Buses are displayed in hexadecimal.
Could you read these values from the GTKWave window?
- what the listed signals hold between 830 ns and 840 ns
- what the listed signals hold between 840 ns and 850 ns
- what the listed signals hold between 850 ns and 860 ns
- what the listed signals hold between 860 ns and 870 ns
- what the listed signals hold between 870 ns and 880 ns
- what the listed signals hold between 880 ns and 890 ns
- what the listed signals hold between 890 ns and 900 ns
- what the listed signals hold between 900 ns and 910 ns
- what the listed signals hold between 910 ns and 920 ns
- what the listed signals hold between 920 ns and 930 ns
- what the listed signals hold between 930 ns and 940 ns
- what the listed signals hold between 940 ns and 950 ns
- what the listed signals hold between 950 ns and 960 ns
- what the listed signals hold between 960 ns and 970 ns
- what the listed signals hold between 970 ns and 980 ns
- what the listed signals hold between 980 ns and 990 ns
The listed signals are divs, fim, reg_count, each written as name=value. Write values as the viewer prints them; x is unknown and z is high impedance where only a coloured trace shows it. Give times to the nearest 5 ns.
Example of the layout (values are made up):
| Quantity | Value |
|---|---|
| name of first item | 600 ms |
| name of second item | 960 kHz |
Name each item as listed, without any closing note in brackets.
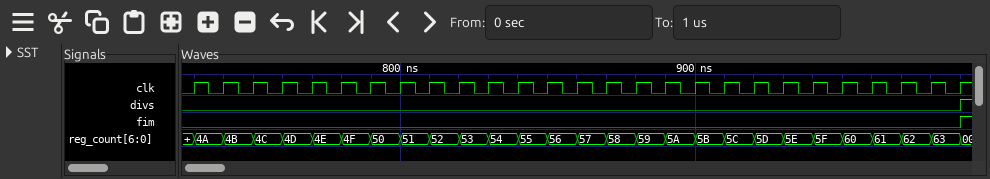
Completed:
| Quantity | Value |
|---|---|
| what the listed signals hold between 830 ns and 840 ns | divs=0, fim=0, reg_count=54 |
| what the listed signals hold between 840 ns and 850 ns | divs=0, fim=0, reg_count=55 |
| what the listed signals hold between 850 ns and 860 ns | divs=0, fim=0, reg_count=56 |
| what the listed signals hold between 860 ns and 870 ns | divs=0, fim=0, reg_count=57 |
| what the listed signals hold between 870 ns and 880 ns | divs=0, fim=0, reg_count=58 |
| what the listed signals hold between 880 ns and 890 ns | divs=0, fim=0, reg_count=59 |
| what the listed signals hold between 890 ns and 900 ns | divs=0, fim=0, reg_count=5A |
| what the listed signals hold between 900 ns and 910 ns | divs=0, fim=0, reg_count=5B |
| what the listed signals hold between 910 ns and 920 ns | divs=0, fim=0, reg_count=5C |
| what the listed signals hold between 920 ns and 930 ns | divs=0, fim=0, reg_count=5D |
| what the listed signals hold between 930 ns and 940 ns | divs=0, fim=0, reg_count=5E |
| what the listed signals hold between 940 ns and 950 ns | divs=0, fim=0, reg_count=5F |
| what the listed signals hold between 950 ns and 960 ns | divs=0, fim=0, reg_count=60 |
| what the listed signals hold between 960 ns and 970 ns | divs=0, fim=0, reg_count=61 |
| what the listed signals hold between 970 ns and 980 ns | divs=0, fim=0, reg_count=62 |
| what the listed signals hold between 980 ns and 990 ns | divs=0, fim=0, reg_count=63 |
